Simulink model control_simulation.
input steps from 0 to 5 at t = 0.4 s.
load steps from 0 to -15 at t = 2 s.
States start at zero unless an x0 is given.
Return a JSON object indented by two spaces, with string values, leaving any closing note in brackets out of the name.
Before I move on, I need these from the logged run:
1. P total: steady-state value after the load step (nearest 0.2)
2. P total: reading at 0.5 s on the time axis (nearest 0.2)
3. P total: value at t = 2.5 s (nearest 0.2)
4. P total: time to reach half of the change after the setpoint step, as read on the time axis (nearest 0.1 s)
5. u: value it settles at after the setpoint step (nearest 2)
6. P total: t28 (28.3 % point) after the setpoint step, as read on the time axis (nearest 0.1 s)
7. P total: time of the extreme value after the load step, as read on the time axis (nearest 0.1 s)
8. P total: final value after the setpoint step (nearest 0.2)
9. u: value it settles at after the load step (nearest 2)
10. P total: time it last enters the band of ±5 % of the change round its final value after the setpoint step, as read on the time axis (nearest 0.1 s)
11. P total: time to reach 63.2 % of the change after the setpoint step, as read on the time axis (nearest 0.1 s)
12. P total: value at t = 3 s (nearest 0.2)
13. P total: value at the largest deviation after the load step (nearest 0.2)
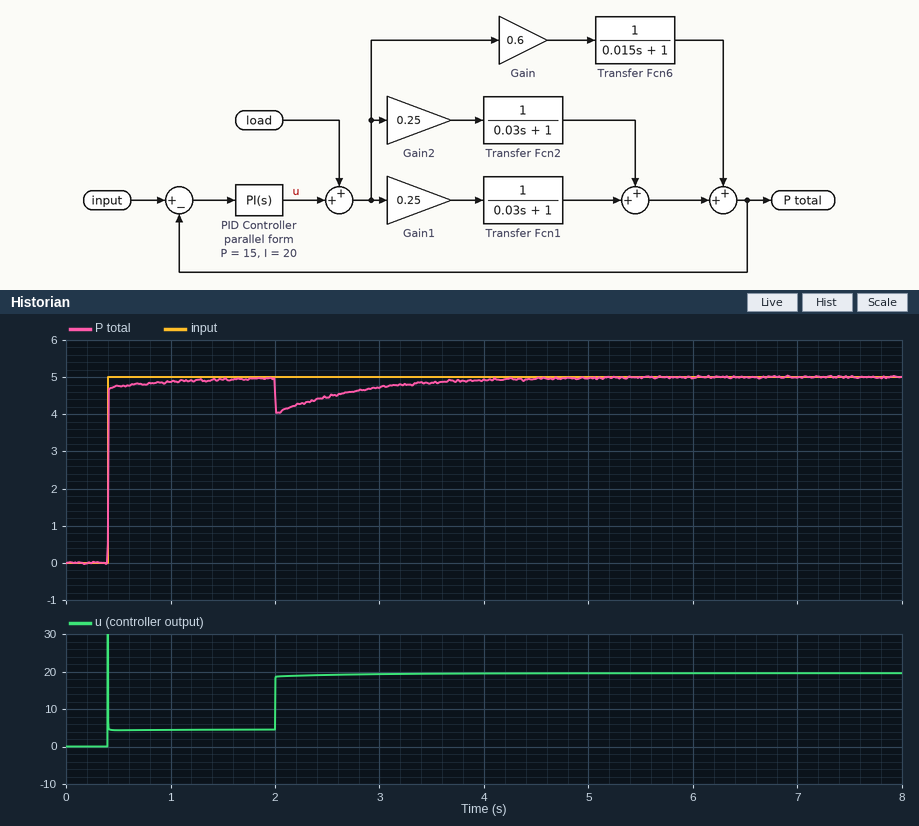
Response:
{
  "P total: steady-state value after the load step": "5.0",
  "P total: reading at 0.5 s on the time axis": "4.8",
  "P total: value at t = 2.5 s": "4.4",
  "P total: time to reach half of the change after the setpoint step, as read on the time axis": "0.4 s",
  "u: value it settles at after the setpoint step": "4",
  "P total: t28 (28.3 % point) after the setpoint step, as read on the time axis": "0.4 s",
  "P total: time of the extreme value after the load step, as read on the time axis": "2.0 s",
  "P total: final value after the setpoint step": "5.0",
  "u: value it settles at after the load step": "20",
  "P total: time it last enters the band of ±5 % of the change round its final value after the setpoint step, as read on the time axis": "0.5 s",
  "P total: time to reach 63.2 % of the change after the setpoint step, as read on the time axis": "0.4 s",
  "P total: value at t = 3 s": "4.8",
  "P total: value at the largest deviation after the load step": "4.0"
}
